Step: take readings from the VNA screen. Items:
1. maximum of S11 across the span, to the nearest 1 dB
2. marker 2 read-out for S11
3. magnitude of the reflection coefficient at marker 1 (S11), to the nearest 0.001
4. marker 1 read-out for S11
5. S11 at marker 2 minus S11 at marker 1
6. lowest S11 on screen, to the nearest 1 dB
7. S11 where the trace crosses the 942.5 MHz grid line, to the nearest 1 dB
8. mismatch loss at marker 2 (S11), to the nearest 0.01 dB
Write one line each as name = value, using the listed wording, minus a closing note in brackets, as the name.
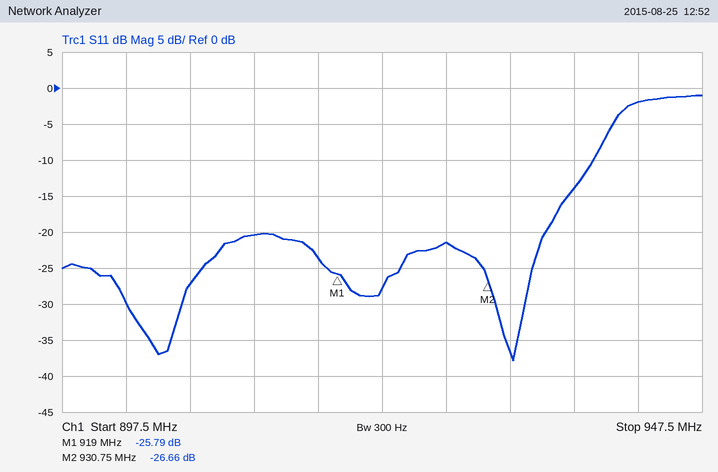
maximum of S11 across the span, to the nearest 1 dB = -1 dB
marker 2 read-out for S11 = -26.66 dB
magnitude of the reflection coefficient at marker 1 (S11), to the nearest 0.001 = 0.051
marker 1 read-out for S11 = -25.79 dB
S11 at marker 2 minus S11 at marker 1 = -0.87 dB
lowest S11 on screen, to the nearest 1 dB = -38 dB
S11 where the trace crosses the 942.5 MHz grid line, to the nearest 1 dB = -2 dB
mismatch loss at marker 2 (S11), to the nearest 0.01 dB = 0.01 dB
